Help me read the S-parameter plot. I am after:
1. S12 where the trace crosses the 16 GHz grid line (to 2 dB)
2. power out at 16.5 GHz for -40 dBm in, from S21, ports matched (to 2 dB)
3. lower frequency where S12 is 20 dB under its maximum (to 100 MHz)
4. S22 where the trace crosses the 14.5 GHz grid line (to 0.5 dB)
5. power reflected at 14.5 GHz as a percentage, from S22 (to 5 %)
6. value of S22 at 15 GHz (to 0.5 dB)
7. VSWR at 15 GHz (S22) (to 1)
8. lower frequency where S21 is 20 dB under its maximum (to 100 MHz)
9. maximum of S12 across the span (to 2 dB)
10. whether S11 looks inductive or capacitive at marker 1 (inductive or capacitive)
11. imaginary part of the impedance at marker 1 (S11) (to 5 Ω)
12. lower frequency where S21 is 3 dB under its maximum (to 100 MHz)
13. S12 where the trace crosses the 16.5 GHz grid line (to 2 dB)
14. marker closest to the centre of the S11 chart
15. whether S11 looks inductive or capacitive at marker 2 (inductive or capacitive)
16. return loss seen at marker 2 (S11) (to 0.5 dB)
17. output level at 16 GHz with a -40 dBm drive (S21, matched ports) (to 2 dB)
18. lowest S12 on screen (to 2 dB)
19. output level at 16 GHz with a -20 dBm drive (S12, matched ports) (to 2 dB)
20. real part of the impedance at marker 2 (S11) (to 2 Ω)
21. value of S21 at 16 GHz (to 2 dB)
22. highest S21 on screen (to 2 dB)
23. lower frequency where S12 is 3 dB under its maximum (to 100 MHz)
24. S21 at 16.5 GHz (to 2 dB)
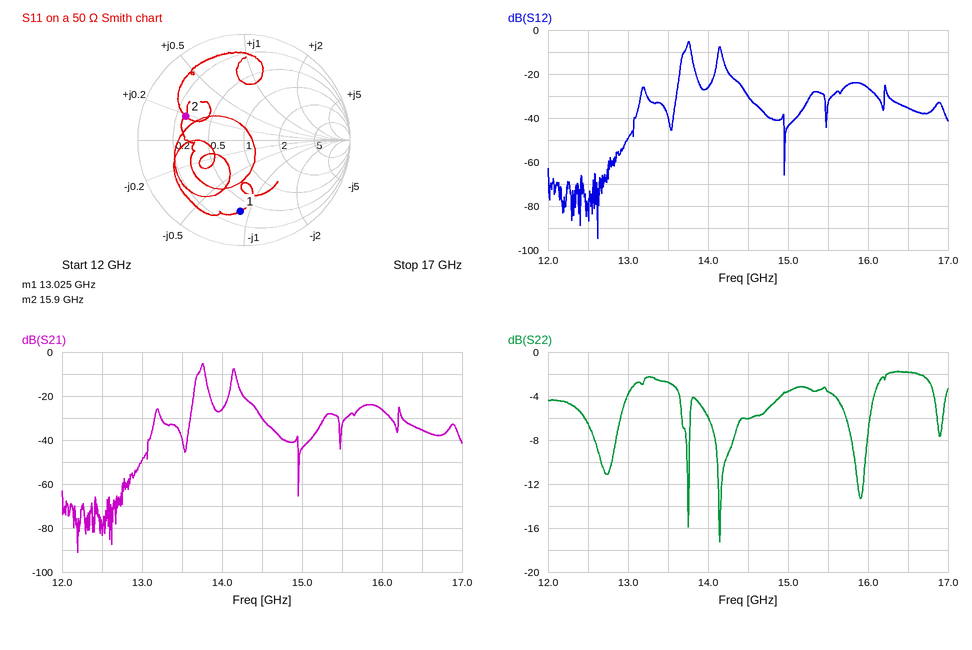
-26 dB
-76 dBm
13.6 GHz
-6.0 dB
25 %
-3.5 dB
5
13.6 GHz
-6 dB
capacitive
-45 Ω
13.7 GHz
-36 dB
marker 2
inductive
4.5 dB
-66 dBm
-94 dB
-46 dBm
14 Ω
-26 dB
-6 dB
13.7 GHz
-36 dB
